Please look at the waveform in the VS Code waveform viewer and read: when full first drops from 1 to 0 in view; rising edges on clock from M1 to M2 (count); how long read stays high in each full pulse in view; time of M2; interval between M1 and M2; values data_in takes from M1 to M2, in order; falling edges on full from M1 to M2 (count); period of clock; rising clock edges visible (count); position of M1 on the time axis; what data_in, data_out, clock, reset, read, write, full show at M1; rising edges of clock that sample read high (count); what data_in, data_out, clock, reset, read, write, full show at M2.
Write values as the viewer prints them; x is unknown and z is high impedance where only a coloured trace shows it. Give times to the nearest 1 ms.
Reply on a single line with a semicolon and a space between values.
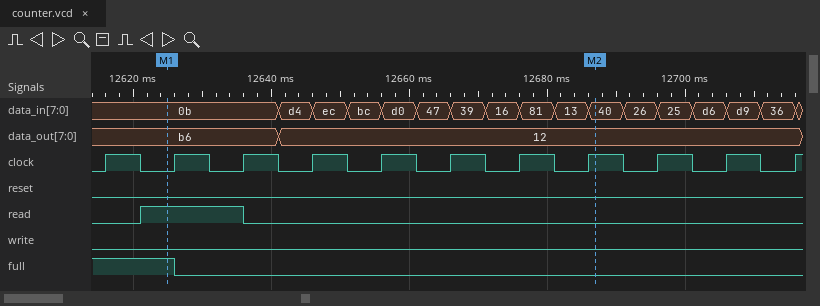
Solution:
12626 ms; 7; 15 ms; 12687 ms; 62 ms; 0b, d4, ec, bc, d0, 47, 39, 16, 81, 13, 40; 1; 10 ms; 11; 12625 ms; data_in=0b, data_out=b6, clock=0, reset=0, read=1, write=0, full=1; 2; data_in=40, data_out=12, clock=1, reset=0, read=0, write=0, full=0
